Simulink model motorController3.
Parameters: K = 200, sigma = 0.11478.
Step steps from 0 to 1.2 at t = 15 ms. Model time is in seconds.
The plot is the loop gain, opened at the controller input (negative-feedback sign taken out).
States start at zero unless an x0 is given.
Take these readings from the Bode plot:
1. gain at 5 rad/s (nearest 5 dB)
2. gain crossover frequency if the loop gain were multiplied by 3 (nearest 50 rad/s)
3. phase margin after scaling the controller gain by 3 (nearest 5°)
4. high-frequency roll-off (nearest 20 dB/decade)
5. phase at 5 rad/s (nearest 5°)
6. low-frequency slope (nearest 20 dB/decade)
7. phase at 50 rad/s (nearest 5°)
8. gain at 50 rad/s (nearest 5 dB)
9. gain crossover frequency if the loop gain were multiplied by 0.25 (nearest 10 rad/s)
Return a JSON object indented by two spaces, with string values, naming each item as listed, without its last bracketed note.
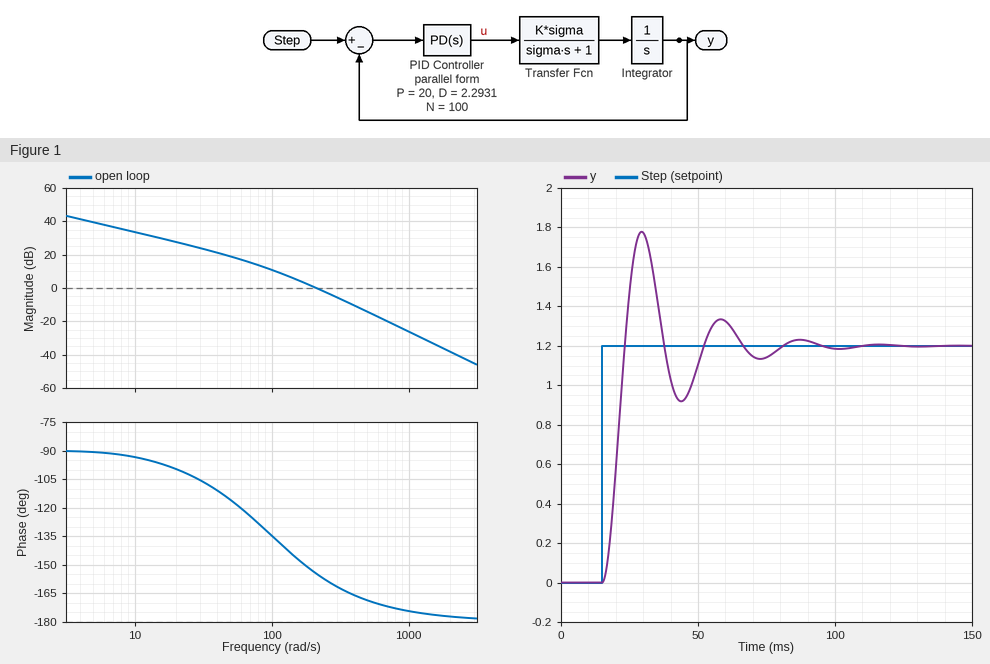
{
  "gain at 5 rad/s": "40 dB",
  "gain crossover frequency if the loop gain were multiplied by 3": "400 rad/s",
  "phase margin after scaling the controller gain by 3": "15°",
  "high-frequency roll-off": "-40 dB/decade",
  "phase at 5 rad/s": "-90°",
  "low-frequency slope": "-20 dB/decade",
  "phase at 50 rad/s": "-115°",
  "gain at 50 rad/s": "20 dB",
  "gain crossover frequency if the loop gain were multiplied by 0.25": "90 rad/s"
}
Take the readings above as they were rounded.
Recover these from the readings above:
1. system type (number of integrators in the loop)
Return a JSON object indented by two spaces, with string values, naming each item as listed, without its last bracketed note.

{
  "system type": "1"
}
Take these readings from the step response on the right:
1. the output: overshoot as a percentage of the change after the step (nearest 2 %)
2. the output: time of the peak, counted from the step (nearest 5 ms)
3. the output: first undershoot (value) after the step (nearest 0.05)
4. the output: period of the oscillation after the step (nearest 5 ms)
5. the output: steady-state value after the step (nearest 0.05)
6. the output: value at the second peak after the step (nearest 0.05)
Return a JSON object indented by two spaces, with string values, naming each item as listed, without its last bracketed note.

{
  "the output: overshoot as a percentage of the change after the step": "48 %",
  "the output: time of the peak, counted from the step": "15 ms",
  "the output: first undershoot (value) after the step": "0.90",
  "the output: period of the oscillation after the step": "30 ms",
  "the output: steady-state value after the step": "1.20",
  "the output: value at the second peak after the step": "1.35"
}
